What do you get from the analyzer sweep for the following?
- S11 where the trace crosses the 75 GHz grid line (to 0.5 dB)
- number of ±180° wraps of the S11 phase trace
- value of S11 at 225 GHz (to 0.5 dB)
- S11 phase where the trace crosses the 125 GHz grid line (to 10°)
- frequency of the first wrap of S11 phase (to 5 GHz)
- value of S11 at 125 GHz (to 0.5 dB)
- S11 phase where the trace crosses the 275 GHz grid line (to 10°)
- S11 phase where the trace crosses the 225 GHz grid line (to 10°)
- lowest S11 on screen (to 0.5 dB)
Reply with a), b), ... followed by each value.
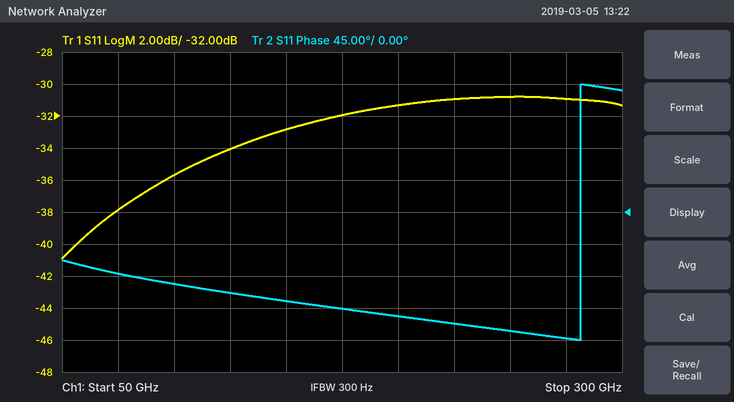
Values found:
a) -38.0 dB
b) 1
c) -31.0 dB
d) -110°
e) 280 GHz
f) -34.0 dB
g) -180°
h) -160°
i) -41.0 dB
